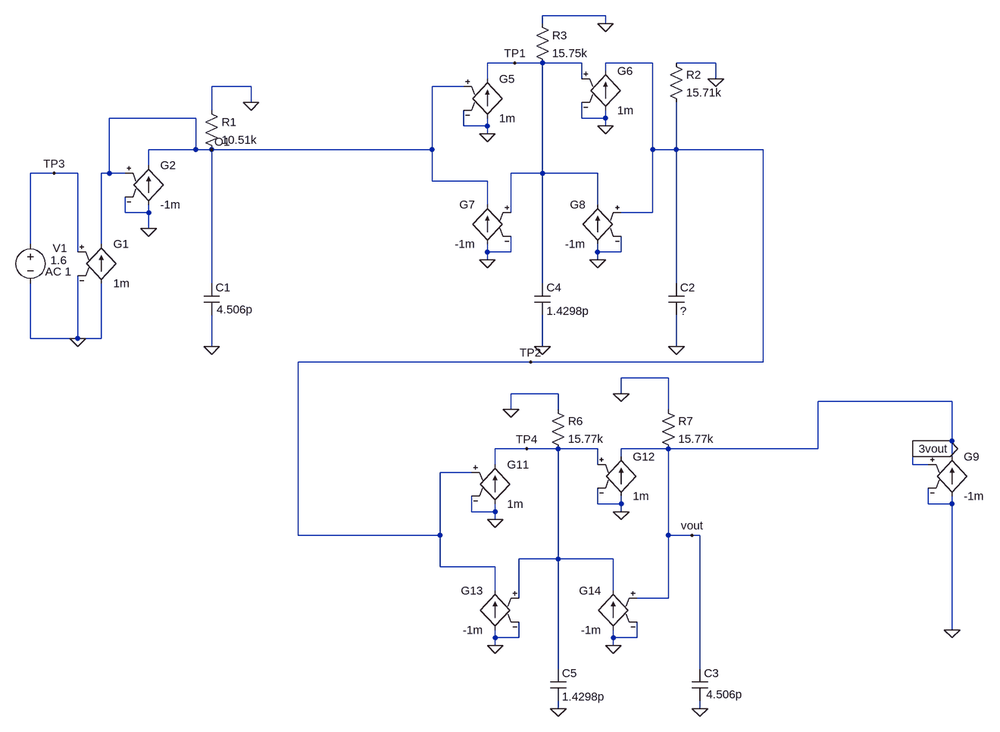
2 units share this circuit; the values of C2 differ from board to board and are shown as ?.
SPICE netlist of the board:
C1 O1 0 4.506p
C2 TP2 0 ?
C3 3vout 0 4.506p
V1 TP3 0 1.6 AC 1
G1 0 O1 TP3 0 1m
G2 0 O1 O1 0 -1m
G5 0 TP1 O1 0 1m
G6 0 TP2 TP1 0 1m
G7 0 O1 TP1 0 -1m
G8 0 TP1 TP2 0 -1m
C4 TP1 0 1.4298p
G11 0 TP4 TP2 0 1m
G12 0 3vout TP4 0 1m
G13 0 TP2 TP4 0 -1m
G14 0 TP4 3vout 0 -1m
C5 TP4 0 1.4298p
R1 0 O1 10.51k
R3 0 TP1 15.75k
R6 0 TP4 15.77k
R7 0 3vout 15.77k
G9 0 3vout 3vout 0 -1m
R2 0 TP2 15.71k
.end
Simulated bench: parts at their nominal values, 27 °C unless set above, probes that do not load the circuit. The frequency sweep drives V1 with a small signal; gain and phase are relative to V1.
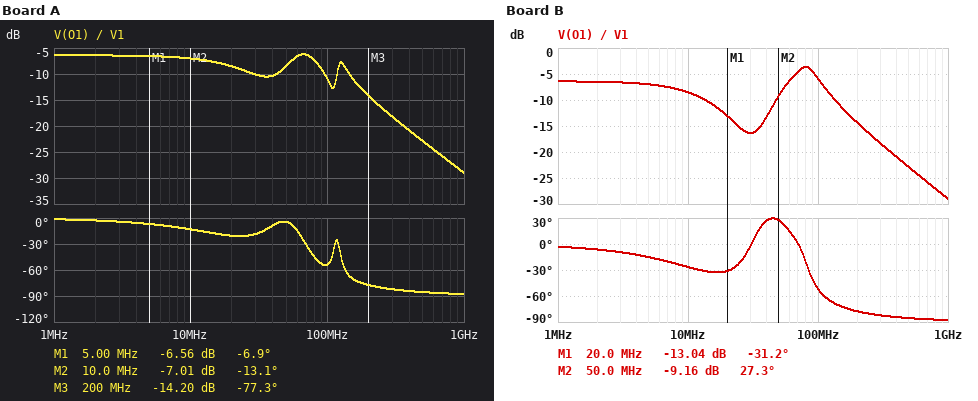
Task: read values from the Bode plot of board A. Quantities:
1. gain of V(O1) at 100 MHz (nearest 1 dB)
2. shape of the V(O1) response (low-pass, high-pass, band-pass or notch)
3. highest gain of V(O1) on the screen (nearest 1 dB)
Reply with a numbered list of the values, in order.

1. -11 dB
2. low-pass
3. -6 dB
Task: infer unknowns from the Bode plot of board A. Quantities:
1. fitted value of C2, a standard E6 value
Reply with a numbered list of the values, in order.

1. 3.3 pF
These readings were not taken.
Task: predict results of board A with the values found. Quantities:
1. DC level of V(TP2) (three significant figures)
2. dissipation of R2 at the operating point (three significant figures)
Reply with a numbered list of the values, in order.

1. 718 mV
2. 32.8 µW
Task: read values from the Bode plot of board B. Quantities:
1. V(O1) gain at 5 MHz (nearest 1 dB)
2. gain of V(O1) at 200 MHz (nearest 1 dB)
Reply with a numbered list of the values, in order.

1. -7 dB
2. -14 dB
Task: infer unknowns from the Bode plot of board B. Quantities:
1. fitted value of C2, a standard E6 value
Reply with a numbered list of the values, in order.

1. 15 pF
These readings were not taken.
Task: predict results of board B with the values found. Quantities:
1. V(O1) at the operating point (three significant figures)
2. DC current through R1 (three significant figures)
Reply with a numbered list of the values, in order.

1. 766 mV
2. 72.9 µA
